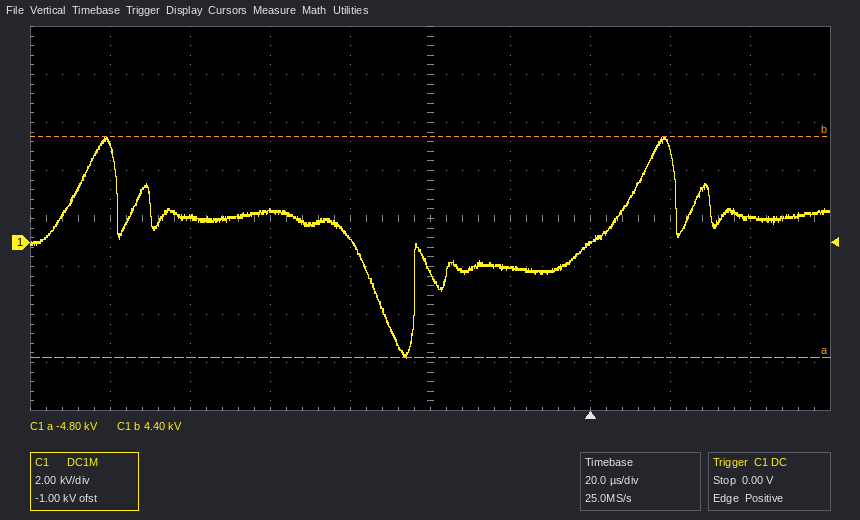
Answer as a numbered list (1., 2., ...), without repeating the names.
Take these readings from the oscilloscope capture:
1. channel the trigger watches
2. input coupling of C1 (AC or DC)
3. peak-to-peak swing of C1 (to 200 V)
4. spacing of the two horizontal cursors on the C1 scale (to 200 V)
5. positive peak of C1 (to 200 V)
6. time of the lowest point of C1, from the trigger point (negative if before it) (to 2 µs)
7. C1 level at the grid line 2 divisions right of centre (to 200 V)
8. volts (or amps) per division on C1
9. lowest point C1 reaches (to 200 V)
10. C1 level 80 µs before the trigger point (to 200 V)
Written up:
1. C1
2. DC
3. 9.2 kV
4. 9.2 kV
5. 4.4 kV
6. -46 µs
7. 0.0 kV
8. 2 kV
9. -4.8 kV
10. 1.2 kV
